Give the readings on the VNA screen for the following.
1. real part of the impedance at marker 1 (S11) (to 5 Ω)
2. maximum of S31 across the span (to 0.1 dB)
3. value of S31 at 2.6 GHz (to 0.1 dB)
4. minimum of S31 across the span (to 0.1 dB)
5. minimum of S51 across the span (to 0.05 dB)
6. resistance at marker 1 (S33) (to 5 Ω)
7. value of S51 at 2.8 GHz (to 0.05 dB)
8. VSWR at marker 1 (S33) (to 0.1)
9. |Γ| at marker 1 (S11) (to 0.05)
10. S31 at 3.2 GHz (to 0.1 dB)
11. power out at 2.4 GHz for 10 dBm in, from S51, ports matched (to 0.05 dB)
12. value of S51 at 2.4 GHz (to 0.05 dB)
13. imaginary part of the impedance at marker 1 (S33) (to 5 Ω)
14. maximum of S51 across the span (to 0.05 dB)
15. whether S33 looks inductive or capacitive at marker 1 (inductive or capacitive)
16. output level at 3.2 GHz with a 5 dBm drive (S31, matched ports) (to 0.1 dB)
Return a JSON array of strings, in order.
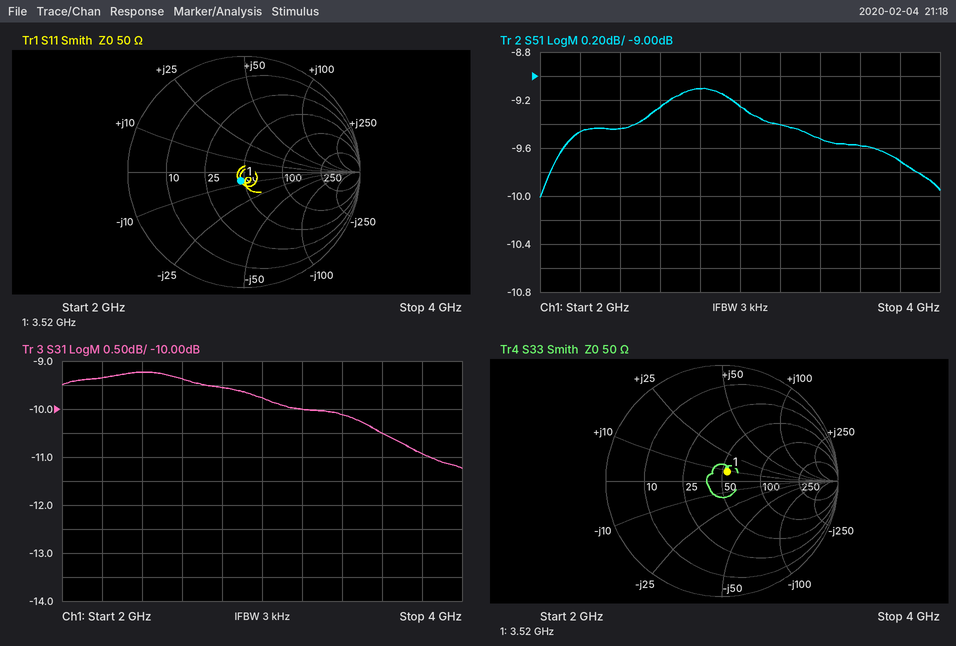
["45 Ω", "-9.2 dB", "-9.4 dB", "-11.2 dB", "-10.00 dB", "55 Ω", "-9.10 dB", "1.2", "0.10", "-10.0 dB", "0.55 dBm", "-9.45 dB", "+10 Ω", "-9.10 dB", "inductive", "-5.0 dBm"]
